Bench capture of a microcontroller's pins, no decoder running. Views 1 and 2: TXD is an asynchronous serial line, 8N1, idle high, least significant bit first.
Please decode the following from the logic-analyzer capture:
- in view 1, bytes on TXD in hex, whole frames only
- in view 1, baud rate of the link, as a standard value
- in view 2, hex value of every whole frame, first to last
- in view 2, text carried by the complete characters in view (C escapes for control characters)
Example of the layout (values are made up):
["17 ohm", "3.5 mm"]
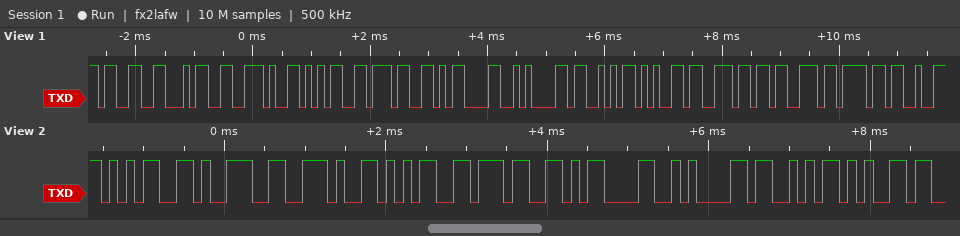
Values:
["0x33 0x34 0x2E 0x35 0x37 0x0D 0x0A 0x53 0x65 0x6E 0x73 0x6F", "9600 baud", "0x35 0x39 0x2E 0x35 0x37 0x0D 0x0A 0x53 0x65", "\"59.57\\r\\nSe\""]
